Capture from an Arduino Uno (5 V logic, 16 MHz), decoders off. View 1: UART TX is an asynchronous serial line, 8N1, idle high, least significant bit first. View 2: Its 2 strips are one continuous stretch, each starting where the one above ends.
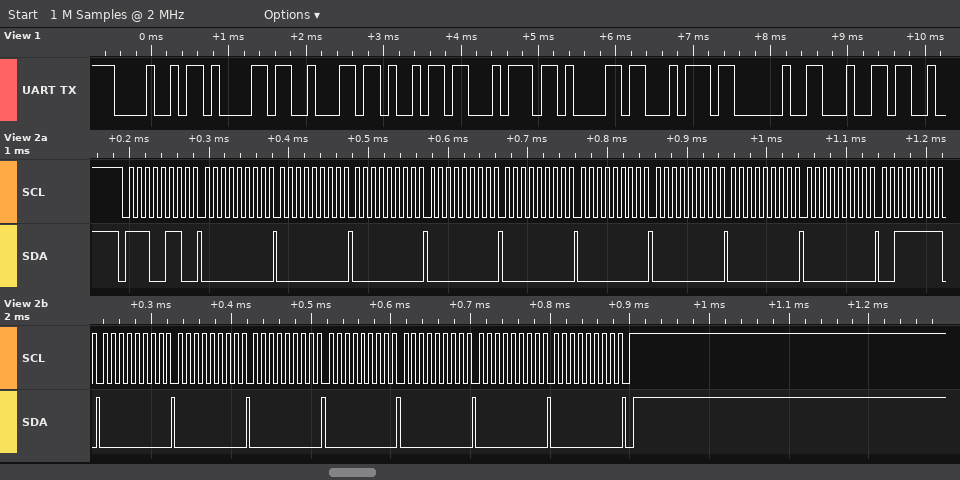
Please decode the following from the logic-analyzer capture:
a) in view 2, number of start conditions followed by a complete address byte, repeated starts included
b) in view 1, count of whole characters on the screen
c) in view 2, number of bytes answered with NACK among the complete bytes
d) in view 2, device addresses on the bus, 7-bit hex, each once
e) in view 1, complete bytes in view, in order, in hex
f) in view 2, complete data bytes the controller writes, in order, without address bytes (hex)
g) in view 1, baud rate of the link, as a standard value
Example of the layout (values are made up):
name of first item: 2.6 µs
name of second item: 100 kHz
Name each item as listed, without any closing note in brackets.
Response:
in view 2, number of start conditions followed by a complete address byte, repeated starts included: 1
in view 1, count of whole characters on the screen: 9
in view 2, number of bytes answered with NACK among the complete bytes: 0
in view 2, device addresses on the bus, 7-bit hex, each once: 0x73
in view 1, complete bytes in view, in order, in hex: 48 61 62 69 74 61 74 20 64
in view 2, complete data bytes the controller writes, in order, without address bytes: 00 00 00 00 00 00 00 00 00 3F 00 00 00 00 00 00 00
in view 1, baud rate of the link, as a standard value: 9600 baud
